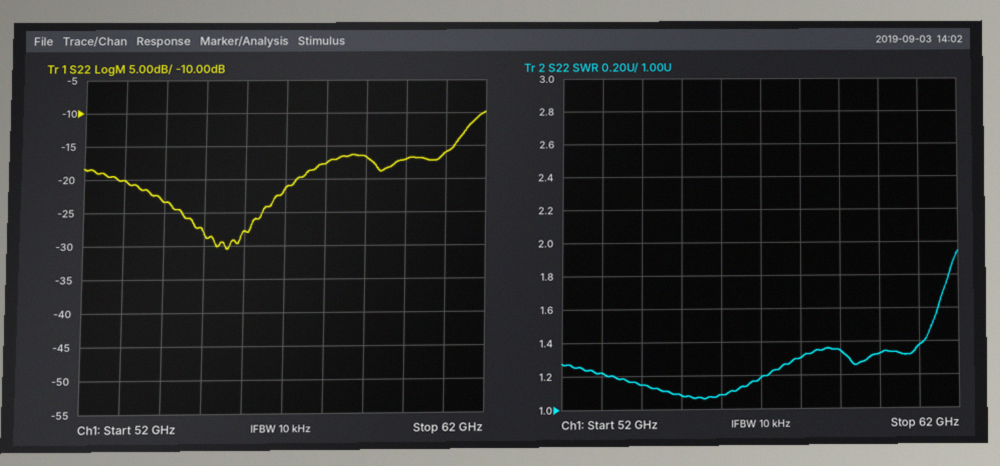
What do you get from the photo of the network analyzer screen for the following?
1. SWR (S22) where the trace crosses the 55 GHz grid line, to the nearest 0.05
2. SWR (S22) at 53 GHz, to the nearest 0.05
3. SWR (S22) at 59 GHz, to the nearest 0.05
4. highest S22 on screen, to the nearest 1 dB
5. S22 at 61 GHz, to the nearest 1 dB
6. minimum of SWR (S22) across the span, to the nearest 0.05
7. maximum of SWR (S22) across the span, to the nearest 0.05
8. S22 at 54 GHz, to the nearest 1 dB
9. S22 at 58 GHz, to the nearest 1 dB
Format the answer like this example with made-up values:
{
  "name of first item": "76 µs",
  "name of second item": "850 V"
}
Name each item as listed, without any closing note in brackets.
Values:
{
  "SWR (S22) where the trace crosses the 55 GHz grid line, to the nearest 0.05": "1.10",
  "SWR (S22) at 53 GHz, to the nearest 0.05": "1.20",
  "SWR (S22) at 59 GHz, to the nearest 0.05": "1.35",
  "highest S22 on screen, to the nearest 1 dB": "-10 dB",
  "S22 at 61 GHz, to the nearest 1 dB": "-16 dB",
  "minimum of SWR (S22) across the span, to the nearest 0.05": "1.05",
  "maximum of SWR (S22) across the span, to the nearest 0.05": "1.95",
  "S22 at 54 GHz, to the nearest 1 dB": "-23 dB",
  "S22 at 58 GHz, to the nearest 1 dB": "-18 dB"
}
